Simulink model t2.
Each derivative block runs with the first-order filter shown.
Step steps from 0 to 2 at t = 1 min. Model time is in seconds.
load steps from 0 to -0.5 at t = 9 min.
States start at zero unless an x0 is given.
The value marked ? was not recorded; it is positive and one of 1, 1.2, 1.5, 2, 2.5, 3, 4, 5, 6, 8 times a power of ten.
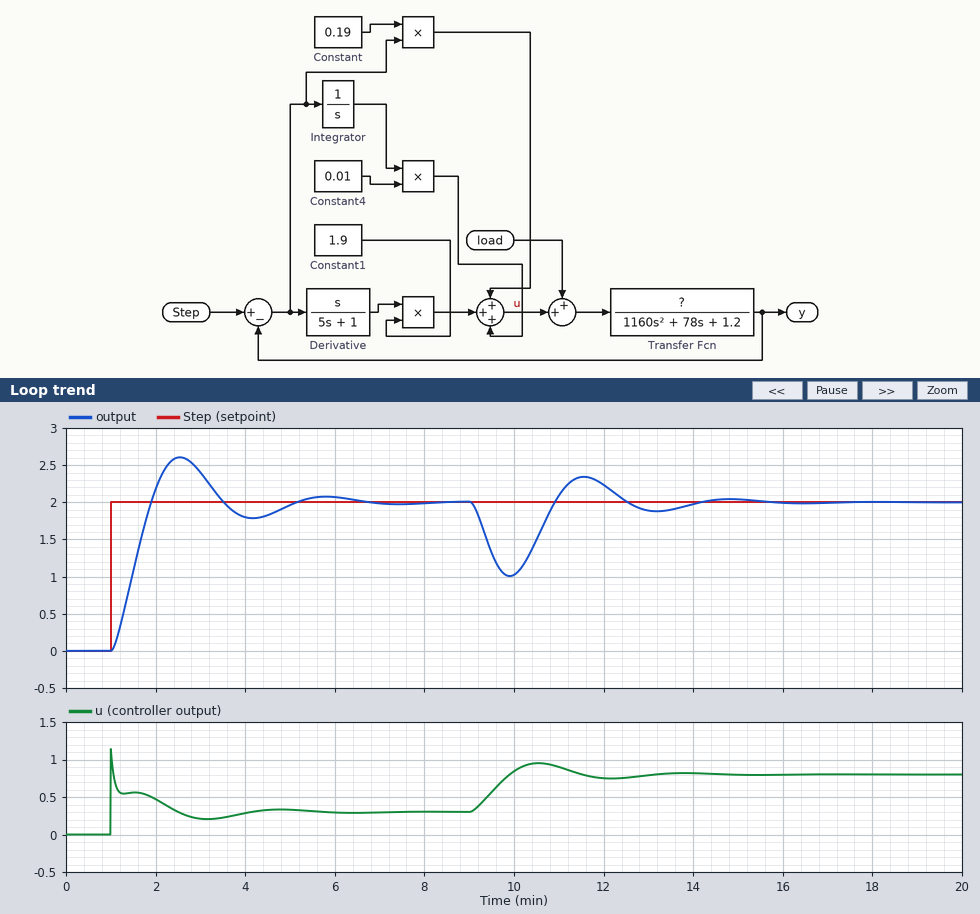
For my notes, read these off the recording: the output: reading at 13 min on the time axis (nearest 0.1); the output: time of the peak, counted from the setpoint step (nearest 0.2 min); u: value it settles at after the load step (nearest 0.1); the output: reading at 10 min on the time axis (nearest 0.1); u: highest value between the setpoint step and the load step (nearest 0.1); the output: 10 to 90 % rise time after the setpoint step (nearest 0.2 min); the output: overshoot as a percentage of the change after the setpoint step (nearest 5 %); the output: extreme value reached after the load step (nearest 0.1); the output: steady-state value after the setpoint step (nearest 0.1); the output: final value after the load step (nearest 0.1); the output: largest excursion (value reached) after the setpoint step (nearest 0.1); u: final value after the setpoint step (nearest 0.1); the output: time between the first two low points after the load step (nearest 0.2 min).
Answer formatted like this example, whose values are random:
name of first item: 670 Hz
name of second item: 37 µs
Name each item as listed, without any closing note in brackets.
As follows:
the output: reading at 13 min on the time axis: 1.9
the output: time of the peak, counted from the setpoint step: 1.6 min
u: value it settles at after the load step: 0.8
the output: reading at 10 min on the time axis: 1.0
u: highest value between the setpoint step and the load step: 1.1
the output: 10 to 90 % rise time after the setpoint step: 0.6 min
the output: overshoot as a percentage of the change after the setpoint step: 30 %
the output: extreme value reached after the load step: 1.0
the output: steady-state value after the setpoint step: 2.0
the output: final value after the load step: 2.0
the output: largest excursion (value reached) after the setpoint step: 2.6
u: final value after the setpoint step: 0.3
the output: time between the first two low points after the load step: 3.2 min
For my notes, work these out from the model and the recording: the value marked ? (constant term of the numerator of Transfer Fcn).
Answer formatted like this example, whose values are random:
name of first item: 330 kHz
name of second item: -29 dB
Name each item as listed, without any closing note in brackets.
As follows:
the value marked ?: 8
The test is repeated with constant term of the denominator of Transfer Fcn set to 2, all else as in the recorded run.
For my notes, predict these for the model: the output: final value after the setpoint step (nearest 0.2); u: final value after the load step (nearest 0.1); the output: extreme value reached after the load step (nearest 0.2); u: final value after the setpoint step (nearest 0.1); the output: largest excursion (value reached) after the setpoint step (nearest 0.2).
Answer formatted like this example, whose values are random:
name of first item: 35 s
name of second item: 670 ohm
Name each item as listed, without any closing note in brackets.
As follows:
the output: final value after the setpoint step: 2.0
u: final value after the load step: 1.0
the output: extreme value reached after the load step: 1.2
u: final value after the setpoint step: 0.5
the output: largest excursion (value reached) after the setpoint step: 2.2
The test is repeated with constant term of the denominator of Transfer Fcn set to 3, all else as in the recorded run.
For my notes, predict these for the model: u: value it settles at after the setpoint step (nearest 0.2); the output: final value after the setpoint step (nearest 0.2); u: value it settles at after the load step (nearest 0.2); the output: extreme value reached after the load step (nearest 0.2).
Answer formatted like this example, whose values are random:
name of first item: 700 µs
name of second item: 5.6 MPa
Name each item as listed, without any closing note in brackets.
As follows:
u: value it settles at after the setpoint step: 0.8
the output: final value after the setpoint step: 2.0
u: value it settles at after the load step: 1.2
the output: extreme value reached after the load step: 1.2
